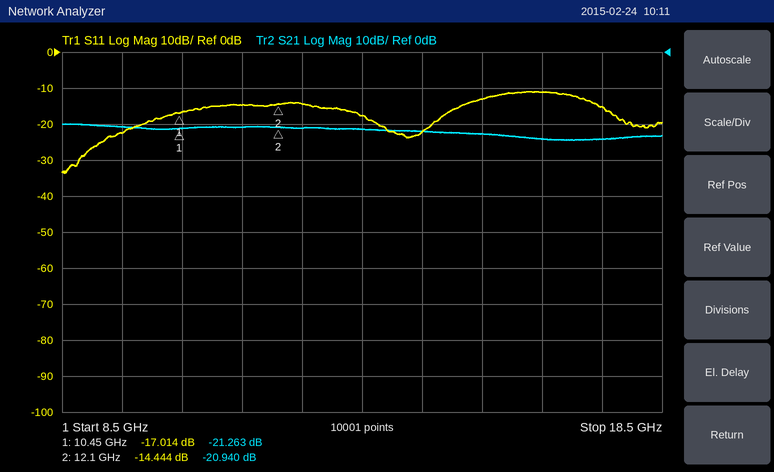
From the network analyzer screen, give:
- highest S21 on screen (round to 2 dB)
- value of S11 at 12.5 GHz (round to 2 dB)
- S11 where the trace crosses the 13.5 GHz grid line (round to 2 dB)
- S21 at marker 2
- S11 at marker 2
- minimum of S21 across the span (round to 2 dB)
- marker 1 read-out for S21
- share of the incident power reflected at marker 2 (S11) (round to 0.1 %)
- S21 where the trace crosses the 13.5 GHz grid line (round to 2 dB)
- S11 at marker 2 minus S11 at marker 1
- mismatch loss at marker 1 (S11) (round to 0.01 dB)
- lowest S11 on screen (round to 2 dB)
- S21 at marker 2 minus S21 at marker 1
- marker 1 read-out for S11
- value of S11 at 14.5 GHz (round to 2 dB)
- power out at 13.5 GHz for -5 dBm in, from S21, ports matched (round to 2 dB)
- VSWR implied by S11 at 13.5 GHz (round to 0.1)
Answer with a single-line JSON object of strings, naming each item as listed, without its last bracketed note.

{"highest S21 on screen": "-20 dB", "value of S11 at 12.5 GHz": "-14 dB", "S11 where the trace crosses the 13.5 GHz grid line": "-18 dB", "S21 at marker 2": "-20.940 dB", "S11 at marker 2": "-14.444 dB", "minimum of S21 across the span": "-24 dB", "marker 1 read-out for S21": "-21.263 dB", "share of the incident power reflected at marker 2 (S11)": "3.6 %", "S21 where the trace crosses the 13.5 GHz grid line": "-22 dB", "S11 at marker 2 minus S11 at marker 1": "2.570 dB", "mismatch loss at marker 1 (S11)": "0.09 dB", "lowest S11 on screen": "-34 dB", "S21 at marker 2 minus S21 at marker 1": "0.323 dB", "marker 1 read-out for S11": "-17.014 dB", "value of S11 at 14.5 GHz": "-22 dB", "power out at 13.5 GHz for -5 dBm in, from S21, ports matched": "-26 dBm", "VSWR implied by S11 at 13.5 GHz": "1.3"}
